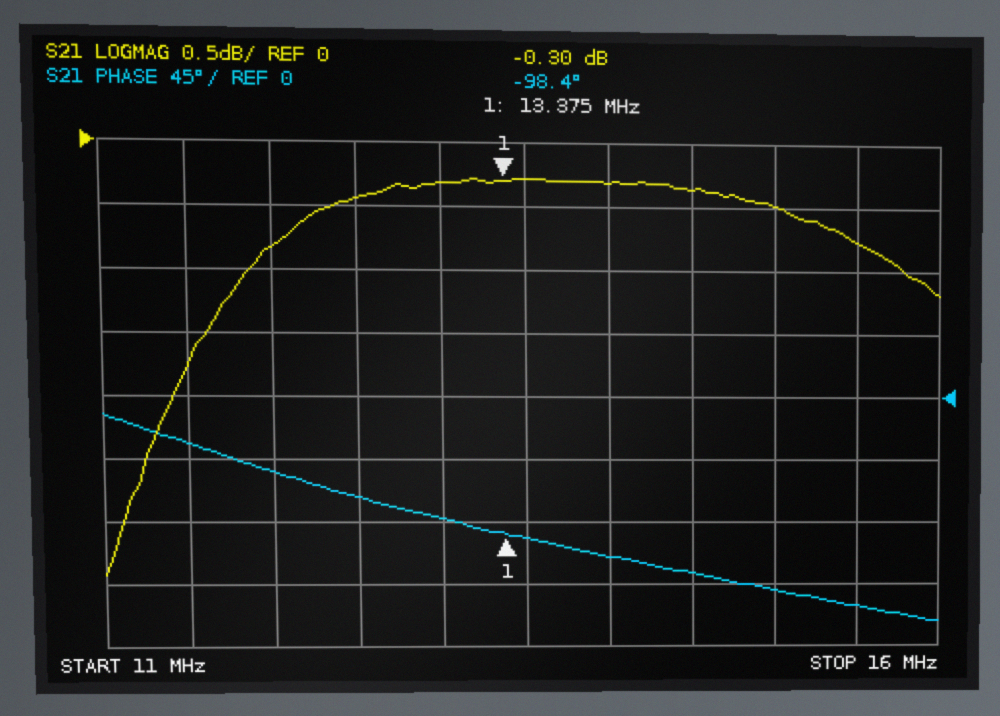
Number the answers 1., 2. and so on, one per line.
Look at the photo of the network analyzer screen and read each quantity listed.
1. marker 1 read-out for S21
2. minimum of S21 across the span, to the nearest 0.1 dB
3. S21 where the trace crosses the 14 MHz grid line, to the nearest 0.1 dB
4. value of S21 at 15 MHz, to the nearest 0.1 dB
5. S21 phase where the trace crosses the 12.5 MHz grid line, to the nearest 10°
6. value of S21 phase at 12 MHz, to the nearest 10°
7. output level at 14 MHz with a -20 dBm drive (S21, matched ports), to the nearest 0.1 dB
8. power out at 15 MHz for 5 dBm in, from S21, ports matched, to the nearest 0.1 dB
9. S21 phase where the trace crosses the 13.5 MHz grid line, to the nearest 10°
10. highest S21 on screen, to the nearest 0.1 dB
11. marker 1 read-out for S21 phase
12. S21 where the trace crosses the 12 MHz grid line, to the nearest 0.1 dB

1. -0.30 dB
2. -3.4 dB
3. -0.3 dB
4. -0.5 dB
5. -70°
6. -50°
7. -20.3 dBm
8. 4.5 dBm
9. -100°
10. -0.3 dB
11. -98.4°
12. -0.8 dB
